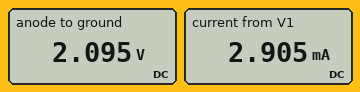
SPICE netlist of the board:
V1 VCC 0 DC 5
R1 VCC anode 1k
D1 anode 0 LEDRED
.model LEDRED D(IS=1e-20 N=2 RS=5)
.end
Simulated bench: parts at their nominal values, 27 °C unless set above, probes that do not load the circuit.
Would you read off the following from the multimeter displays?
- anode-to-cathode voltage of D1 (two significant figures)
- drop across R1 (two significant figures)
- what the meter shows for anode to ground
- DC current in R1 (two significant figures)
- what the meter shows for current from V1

2.1 V
2.9 V
2.095 V
2.9 mA
2.905 mA
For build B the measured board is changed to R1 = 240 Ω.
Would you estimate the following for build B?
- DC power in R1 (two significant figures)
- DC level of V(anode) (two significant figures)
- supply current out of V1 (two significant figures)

32 mW
2.2 V
12 mA
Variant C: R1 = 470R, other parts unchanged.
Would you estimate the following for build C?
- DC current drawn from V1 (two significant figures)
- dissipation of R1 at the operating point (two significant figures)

6.1 mA
17 mW
